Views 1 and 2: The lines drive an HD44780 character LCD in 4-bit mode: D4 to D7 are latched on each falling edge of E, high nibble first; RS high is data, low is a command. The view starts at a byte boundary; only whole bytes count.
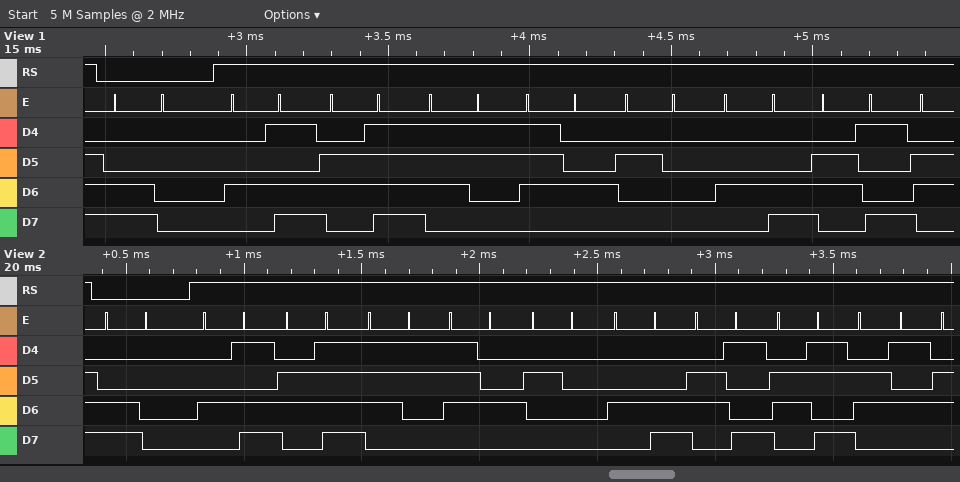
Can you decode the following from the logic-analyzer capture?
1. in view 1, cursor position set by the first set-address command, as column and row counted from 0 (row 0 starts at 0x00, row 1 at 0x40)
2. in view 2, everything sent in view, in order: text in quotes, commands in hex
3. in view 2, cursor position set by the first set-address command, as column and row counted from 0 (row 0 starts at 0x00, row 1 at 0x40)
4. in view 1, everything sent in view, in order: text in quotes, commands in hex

column 0, row 1
0xC0 "Most Like"
column 0, row 1
0xC0 "Most Li"
